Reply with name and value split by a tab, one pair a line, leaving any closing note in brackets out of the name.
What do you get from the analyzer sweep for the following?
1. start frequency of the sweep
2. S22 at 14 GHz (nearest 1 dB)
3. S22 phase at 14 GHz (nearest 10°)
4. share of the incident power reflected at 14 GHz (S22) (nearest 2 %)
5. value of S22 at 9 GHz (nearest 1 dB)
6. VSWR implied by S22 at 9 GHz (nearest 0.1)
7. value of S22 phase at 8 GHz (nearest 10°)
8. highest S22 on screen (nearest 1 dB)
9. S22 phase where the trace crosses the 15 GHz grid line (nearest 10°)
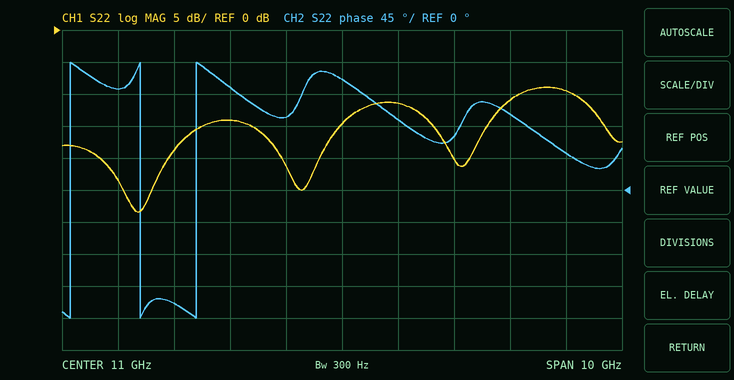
start frequency of the sweep	6 GHz
S22 at 14 GHz	-11 dB
S22 phase at 14 GHz	110°
share of the incident power reflected at 14 GHz (S22)	8 %
value of S22 at 9 GHz	-14 dB
VSWR implied by S22 at 9 GHz	1.5
value of S22 phase at 8 GHz	-160°
highest S22 on screen	-9 dB
S22 phase where the trace crosses the 15 GHz grid line	50°
